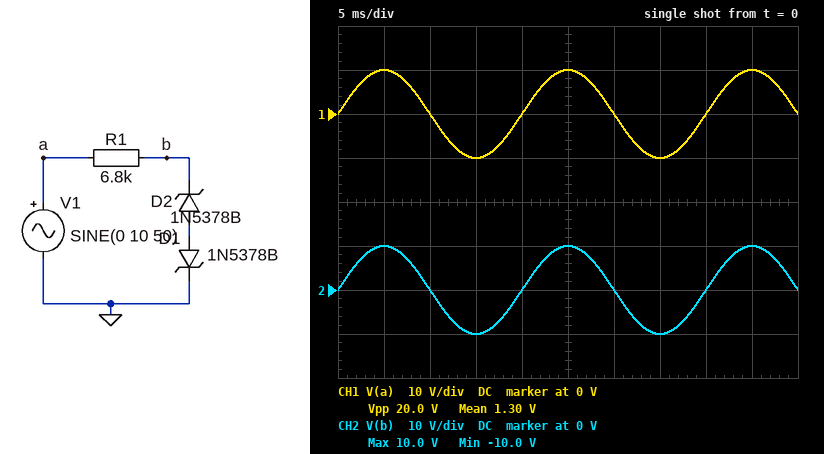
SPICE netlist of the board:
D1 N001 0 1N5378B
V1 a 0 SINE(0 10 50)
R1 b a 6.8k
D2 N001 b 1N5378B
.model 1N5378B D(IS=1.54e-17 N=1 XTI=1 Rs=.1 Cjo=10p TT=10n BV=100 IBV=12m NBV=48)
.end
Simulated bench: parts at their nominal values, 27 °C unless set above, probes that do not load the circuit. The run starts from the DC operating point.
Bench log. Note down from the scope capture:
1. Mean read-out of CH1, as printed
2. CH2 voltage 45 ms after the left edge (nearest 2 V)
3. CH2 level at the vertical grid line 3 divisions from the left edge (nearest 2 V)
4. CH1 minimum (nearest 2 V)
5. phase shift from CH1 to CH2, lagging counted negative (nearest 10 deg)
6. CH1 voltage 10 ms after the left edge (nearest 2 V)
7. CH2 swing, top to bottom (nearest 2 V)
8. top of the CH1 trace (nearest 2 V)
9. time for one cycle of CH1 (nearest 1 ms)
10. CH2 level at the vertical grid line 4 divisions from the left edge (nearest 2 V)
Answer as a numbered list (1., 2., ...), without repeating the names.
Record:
1. 1.30 V
2. 10 V
3. -10 V
4. -10 V
5. 0 deg
6. 0 V
7. 20 V
8. 10 V
9. 20 ms
10. 0 V
